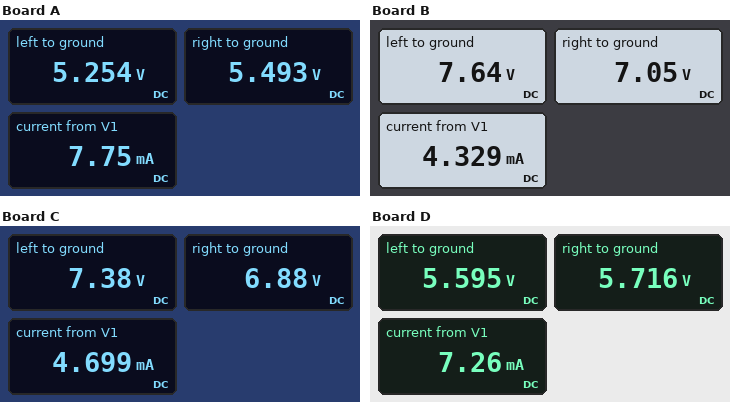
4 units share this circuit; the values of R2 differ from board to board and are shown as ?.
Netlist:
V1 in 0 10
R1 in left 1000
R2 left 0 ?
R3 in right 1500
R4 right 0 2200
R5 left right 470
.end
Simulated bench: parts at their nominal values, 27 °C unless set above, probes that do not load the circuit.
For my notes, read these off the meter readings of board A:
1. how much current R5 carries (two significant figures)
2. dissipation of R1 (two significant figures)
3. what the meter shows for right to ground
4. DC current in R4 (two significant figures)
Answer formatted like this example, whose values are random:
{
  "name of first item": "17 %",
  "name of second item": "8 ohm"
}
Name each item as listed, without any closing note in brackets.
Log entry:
{
  "how much current R5 carries": "510 µA",
  "dissipation of R1": "23 mW",
  "what the meter shows for right to ground": "5.493 V",
  "DC current in R4": "2.5 mA"
}
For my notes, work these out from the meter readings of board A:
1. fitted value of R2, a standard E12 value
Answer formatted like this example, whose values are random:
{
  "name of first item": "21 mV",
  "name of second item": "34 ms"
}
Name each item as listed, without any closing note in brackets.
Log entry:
{
  "fitted value of R2, a standard E12 value": "1 kΩ"
}
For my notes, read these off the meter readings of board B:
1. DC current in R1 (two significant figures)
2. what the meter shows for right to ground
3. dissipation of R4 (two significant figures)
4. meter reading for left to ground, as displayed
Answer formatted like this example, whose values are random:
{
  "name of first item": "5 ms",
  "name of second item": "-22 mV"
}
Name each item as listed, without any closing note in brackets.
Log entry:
{
  "DC current in R1": "2.4 mA",
  "what the meter shows for right to ground": "7.05 V",
  "dissipation of R4": "23 mW",
  "meter reading for left to ground, as displayed": "7.64 V"
}
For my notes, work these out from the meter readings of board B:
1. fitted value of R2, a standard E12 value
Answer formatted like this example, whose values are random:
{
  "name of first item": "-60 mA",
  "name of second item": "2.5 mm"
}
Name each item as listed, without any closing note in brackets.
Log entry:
{
  "fitted value of R2, a standard E12 value": "6.8 kΩ"
}
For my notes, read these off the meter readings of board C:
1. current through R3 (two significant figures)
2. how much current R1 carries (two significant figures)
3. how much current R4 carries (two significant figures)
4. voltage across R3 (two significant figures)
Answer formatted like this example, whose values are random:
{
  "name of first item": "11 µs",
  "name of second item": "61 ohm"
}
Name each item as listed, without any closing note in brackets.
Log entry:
{
  "current through R3": "2.1 mA",
  "how much current R1 carries": "2.6 mA",
  "how much current R4 carries": "3.1 mA",
  "voltage across R3": "3.1 V"
}
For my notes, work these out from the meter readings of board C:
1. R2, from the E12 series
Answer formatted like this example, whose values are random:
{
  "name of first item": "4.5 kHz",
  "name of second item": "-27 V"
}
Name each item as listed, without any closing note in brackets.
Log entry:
{
  "R2, from the E12 series": "4.7 kΩ"
}
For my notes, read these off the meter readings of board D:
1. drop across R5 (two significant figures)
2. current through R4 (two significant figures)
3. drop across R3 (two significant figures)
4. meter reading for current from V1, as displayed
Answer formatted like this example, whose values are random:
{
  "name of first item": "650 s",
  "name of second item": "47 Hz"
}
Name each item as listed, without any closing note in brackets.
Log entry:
{
  "drop across R5": "120 mV",
  "current through R4": "2.6 mA",
  "drop across R3": "4.3 V",
  "meter reading for current from V1, as displayed": "7.26 mA"
}
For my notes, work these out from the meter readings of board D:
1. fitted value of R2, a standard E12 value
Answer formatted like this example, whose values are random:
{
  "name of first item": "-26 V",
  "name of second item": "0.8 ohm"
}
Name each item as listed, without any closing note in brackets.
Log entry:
{
  "fitted value of R2, a standard E12 value": "1.2 kΩ"
}
